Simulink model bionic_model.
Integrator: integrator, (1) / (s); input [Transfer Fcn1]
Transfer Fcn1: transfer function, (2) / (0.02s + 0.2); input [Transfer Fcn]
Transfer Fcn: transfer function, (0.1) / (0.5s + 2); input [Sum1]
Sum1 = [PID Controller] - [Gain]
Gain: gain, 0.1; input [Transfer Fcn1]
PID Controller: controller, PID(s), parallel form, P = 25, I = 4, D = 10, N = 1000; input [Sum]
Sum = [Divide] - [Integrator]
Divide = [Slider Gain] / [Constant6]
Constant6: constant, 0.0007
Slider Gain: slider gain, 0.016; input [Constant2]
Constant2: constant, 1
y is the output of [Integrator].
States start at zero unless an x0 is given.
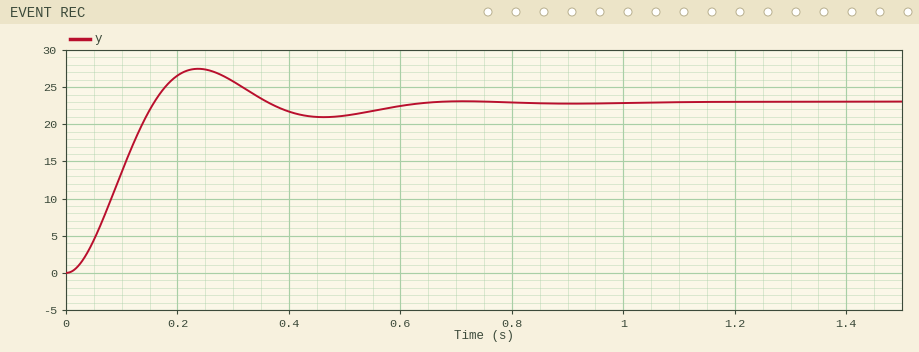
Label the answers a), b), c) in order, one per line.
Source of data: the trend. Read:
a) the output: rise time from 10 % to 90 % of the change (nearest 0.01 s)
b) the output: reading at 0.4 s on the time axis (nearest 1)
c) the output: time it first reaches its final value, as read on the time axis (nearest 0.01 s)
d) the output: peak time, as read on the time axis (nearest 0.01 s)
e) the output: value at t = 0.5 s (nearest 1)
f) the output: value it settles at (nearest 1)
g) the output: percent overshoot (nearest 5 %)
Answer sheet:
a) 0.11 s
b) 22
c) 0.16 s
d) 0.24 s
e) 21
f) 23
g) 20 %
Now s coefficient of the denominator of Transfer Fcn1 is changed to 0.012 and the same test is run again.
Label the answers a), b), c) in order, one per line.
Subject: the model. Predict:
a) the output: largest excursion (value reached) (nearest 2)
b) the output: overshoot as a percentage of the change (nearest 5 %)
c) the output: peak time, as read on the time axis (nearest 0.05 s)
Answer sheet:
a) 26
b) 10 %
c) 0.20 s
